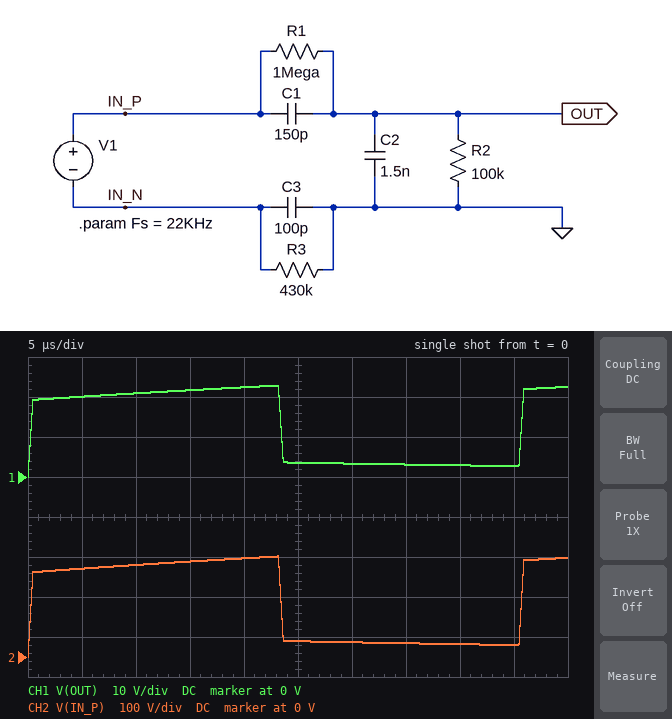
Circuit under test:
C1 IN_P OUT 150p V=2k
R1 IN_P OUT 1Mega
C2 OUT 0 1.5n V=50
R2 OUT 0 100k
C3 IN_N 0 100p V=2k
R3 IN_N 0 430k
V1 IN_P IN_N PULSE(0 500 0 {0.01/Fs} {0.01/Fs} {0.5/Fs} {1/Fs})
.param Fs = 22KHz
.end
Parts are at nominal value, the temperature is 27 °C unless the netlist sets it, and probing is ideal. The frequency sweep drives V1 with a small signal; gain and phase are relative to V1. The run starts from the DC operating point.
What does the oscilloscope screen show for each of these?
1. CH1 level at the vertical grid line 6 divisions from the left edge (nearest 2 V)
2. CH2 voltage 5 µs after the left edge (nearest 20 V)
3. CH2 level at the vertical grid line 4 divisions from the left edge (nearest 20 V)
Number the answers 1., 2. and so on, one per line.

1. 4 V
2. 220 V
3. 240 V
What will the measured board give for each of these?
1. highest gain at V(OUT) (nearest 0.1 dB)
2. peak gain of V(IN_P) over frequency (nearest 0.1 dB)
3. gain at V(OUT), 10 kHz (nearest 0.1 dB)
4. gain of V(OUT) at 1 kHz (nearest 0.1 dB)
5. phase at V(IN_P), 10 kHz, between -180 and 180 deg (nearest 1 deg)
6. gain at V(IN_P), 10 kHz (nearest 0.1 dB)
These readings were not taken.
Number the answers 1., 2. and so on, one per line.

1. -23.7 dB
2. -2.9 dB
3. -27.9 dB
4. -24.2 dB
5. -8 deg
6. -7.1 dB
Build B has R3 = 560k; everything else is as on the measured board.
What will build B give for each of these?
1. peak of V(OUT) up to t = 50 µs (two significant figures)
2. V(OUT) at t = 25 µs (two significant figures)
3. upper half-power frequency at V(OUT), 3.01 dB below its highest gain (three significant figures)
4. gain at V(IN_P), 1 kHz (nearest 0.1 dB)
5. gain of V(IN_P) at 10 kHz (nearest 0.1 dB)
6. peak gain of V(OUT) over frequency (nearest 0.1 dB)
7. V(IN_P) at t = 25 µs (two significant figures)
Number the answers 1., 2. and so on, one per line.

1. 22 V
2. 2.5 V
3. 4.22 kHz
4. -4.2 dB
5. -7.3 dB
6. -24.4 dB
7. 27 V
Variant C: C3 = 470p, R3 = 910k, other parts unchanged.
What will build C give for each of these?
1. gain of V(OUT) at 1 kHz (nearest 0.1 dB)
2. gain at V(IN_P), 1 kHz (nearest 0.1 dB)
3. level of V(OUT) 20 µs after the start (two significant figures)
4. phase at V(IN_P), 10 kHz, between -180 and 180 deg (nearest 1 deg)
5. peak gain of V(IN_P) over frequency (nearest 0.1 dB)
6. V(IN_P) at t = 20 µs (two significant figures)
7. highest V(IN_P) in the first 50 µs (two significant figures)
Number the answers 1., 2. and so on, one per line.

1. -23.5 dB
2. -2.7 dB
3. 35 V
4. 1 deg
5. -2.2 dB
6. 380 V
7. 390 V
